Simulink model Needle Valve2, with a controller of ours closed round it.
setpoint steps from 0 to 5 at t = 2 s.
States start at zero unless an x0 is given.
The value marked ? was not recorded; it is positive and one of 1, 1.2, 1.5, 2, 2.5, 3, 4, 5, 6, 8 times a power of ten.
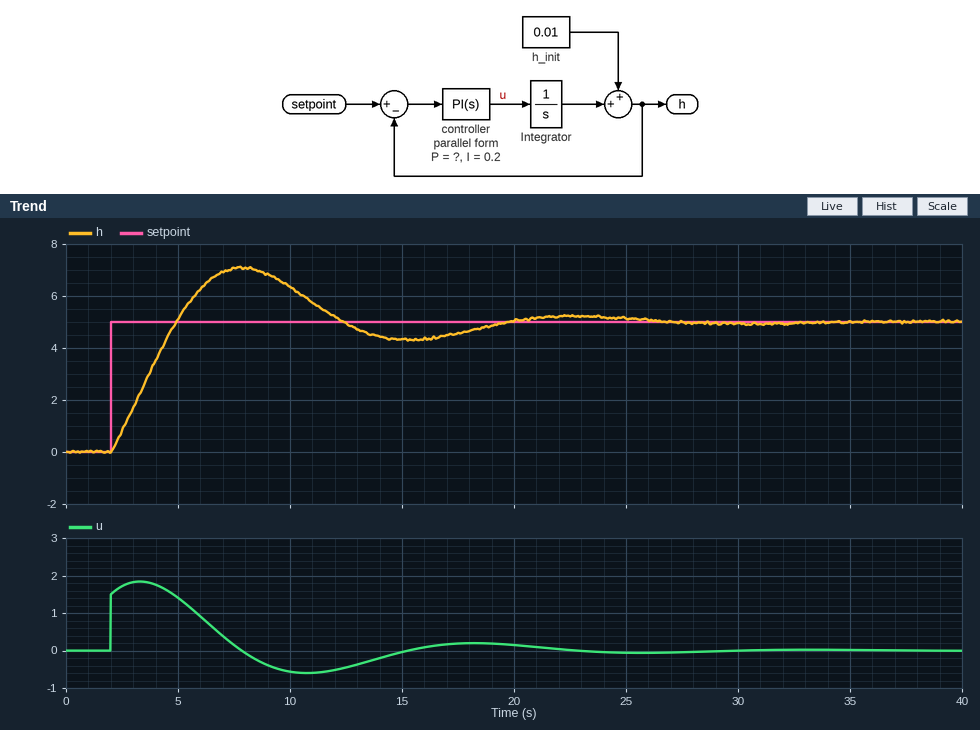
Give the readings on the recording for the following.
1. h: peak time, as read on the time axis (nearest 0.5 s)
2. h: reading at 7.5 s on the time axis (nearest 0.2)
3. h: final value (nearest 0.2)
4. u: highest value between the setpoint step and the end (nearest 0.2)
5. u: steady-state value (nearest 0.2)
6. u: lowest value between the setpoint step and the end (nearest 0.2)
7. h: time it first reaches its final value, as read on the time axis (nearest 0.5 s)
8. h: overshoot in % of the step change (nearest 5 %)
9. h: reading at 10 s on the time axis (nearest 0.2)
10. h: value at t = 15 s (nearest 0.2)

8.0 s
7.0
5.0
1.8
0.0
-0.6
5.0 s
40 %
6.4
4.4
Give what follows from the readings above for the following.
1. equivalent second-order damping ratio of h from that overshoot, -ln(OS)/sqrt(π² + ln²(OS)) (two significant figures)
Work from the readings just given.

0.28
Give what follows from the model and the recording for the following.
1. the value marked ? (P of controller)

0.3
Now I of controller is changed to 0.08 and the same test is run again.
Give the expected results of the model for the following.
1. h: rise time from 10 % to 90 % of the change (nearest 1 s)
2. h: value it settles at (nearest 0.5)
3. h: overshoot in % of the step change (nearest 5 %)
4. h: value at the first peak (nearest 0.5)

3 s
5.0
30 %
6.5
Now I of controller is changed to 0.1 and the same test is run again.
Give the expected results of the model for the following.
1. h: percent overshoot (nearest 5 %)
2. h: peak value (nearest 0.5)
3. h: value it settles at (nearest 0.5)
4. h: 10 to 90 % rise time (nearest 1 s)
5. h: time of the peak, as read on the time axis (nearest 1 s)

30 %
6.5
5.0
3 s
10 s
